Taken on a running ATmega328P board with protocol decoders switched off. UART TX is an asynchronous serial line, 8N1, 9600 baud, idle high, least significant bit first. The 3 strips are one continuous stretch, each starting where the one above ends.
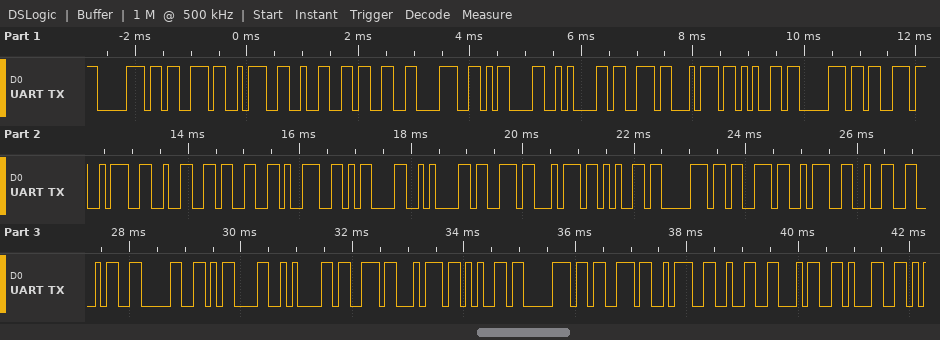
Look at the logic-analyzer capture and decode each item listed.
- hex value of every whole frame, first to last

70 73 3A 32 33 38 0D 0A 73 74 65 70 73 3A 32 33 39 0D 0A 73 74 65 70 73 3A 32 34 30 0D 0A 73 74 65 70 73 3A 32 34 31
